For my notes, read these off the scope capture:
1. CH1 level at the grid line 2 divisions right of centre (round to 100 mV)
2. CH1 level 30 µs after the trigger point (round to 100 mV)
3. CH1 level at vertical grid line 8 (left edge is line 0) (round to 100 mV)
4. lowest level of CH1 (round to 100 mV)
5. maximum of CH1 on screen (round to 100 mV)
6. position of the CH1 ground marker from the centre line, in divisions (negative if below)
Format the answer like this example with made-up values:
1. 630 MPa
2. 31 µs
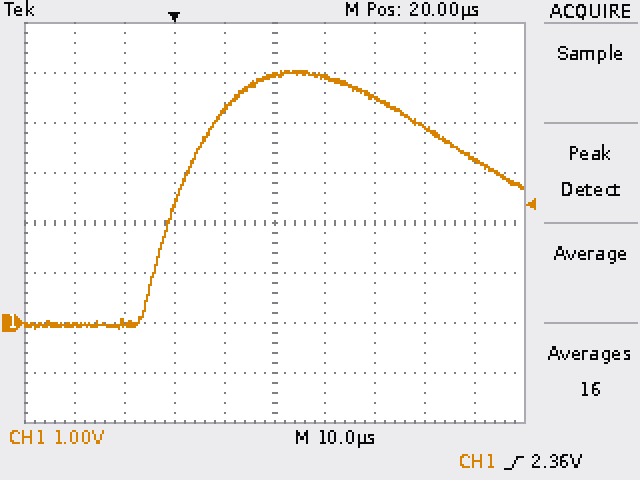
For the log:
1. 4.5 V
2. 4.9 V
3. 3.9 V
4. -100 mV
5. 5.0 V
6. -2.0 div
